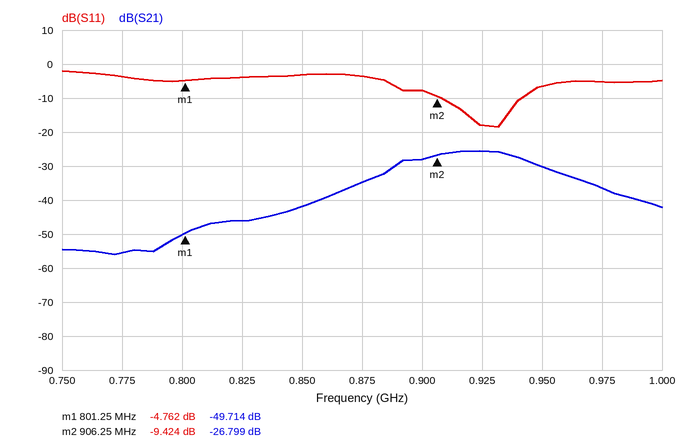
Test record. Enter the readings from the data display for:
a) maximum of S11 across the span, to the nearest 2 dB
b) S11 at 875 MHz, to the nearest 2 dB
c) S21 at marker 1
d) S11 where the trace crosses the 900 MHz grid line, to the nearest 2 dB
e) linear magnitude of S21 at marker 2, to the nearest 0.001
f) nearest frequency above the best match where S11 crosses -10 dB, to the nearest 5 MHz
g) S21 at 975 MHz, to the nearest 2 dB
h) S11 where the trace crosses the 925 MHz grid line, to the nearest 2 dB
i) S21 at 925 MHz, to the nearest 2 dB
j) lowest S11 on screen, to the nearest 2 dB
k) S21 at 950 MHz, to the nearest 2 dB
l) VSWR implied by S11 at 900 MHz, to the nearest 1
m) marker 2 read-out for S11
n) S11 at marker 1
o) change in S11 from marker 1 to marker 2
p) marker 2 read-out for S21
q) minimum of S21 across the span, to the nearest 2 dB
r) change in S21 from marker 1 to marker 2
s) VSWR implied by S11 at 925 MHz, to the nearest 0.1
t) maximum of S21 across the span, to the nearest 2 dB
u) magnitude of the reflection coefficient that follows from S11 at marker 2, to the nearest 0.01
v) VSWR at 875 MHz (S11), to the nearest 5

-2 dB
-4 dB
-49.714 dB
-8 dB
0.046
940 MHz
-36 dB
-18 dB
-26 dB
-18 dB
-30 dB
2
-9.424 dB
-4.762 dB
-4.662 dB
-26.799 dB
-56 dB
22.915 dB
1.3
-26 dB
0.34
5
